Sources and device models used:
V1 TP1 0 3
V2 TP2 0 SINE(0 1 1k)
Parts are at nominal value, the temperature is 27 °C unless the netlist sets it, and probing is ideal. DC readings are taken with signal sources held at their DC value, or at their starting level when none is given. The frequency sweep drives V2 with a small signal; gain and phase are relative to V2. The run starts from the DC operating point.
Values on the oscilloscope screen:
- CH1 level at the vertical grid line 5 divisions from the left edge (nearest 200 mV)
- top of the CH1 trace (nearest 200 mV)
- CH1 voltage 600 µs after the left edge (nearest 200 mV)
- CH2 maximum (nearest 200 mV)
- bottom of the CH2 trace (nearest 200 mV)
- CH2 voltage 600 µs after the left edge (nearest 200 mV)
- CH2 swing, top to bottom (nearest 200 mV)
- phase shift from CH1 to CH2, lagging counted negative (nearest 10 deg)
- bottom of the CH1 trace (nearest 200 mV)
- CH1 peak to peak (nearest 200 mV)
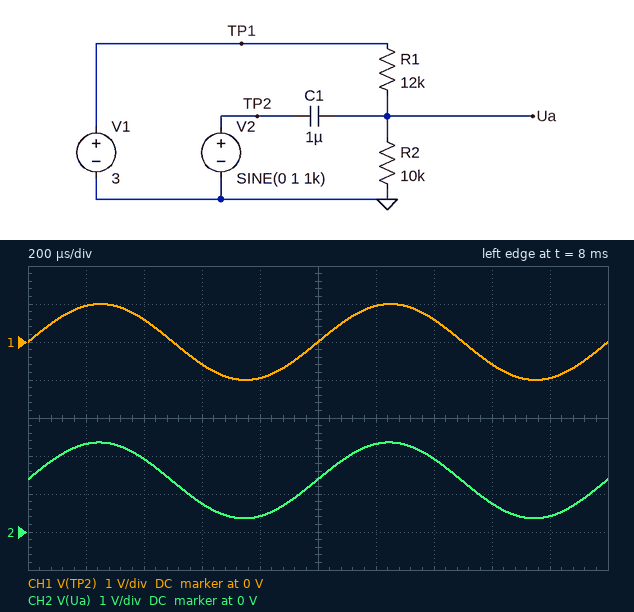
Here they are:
0 V
1.0 V
-600 mV
2.4 V
400 mV
800 mV
2.0 V
0 deg
-1.0 V
2.0 V
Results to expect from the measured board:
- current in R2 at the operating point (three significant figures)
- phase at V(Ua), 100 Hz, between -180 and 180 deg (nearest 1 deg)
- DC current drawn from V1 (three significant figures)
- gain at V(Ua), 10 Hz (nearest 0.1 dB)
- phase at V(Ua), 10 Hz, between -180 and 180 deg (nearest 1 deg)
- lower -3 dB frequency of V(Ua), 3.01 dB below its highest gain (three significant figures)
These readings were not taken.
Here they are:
136 µA
16 deg
136 µA
-9.8 dB
71 deg
29.2 Hz
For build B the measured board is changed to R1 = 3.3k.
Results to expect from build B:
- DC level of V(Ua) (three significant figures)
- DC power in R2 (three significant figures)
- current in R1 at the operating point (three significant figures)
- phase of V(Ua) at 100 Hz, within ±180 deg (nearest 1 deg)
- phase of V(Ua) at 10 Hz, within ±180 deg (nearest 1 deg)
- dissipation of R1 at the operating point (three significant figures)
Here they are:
2.26 V
509 µW
226 µA
33 deg
81 deg
168 µW
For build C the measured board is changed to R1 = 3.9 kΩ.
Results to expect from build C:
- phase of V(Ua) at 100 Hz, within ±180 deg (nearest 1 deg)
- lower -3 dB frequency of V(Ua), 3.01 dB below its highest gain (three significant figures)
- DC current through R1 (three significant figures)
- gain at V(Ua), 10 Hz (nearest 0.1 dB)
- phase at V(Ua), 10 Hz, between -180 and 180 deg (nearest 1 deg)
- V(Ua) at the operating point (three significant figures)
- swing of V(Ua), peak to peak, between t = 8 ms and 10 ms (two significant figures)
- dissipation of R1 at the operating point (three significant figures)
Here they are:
30 deg
56.7 Hz
216 µA
-15.2 dB
80 deg
2.16 V
2.0 V
182 µW
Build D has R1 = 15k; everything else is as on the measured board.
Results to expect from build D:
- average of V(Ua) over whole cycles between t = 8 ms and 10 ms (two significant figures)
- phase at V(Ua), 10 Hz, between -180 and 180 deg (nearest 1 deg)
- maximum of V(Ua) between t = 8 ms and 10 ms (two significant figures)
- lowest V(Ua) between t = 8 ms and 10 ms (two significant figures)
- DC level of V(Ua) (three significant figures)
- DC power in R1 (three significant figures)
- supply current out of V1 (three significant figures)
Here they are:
1.2 V
69 deg
2.2 V
190 mV
1.20 V
216 µW
120 µA
